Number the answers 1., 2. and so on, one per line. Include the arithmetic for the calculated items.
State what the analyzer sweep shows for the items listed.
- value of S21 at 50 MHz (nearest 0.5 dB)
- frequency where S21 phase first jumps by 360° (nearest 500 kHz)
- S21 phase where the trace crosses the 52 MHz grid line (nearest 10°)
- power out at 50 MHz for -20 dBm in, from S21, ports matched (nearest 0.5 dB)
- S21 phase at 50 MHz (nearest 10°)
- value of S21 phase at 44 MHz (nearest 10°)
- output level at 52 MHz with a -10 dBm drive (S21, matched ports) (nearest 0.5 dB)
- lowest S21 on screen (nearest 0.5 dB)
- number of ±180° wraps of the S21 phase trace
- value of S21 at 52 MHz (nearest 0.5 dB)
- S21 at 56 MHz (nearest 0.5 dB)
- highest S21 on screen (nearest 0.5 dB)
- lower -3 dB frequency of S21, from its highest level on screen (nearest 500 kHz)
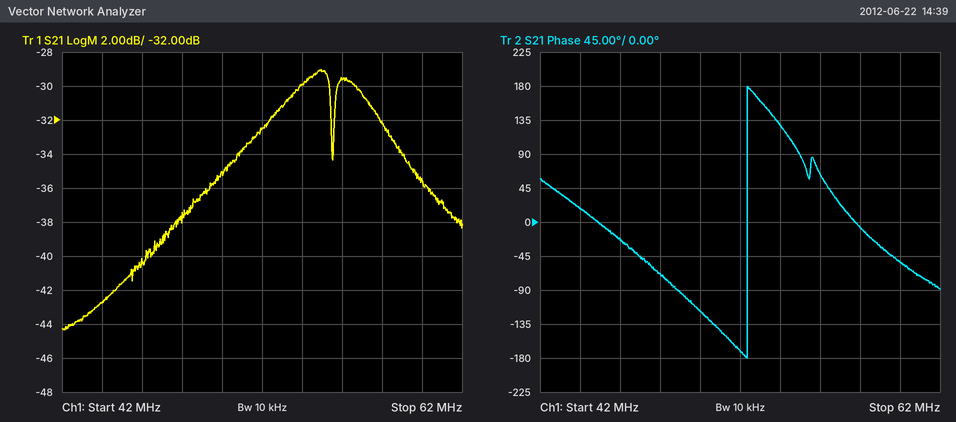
1. -35.0 dB
2. 52.5 MHz
3. -170°
4. -20 dBm + (-35.0 dB) = -55.0 dBm
5. -120°
6. 20°
7. -10 dBm + (-32.5 dB) = -42.5 dBm
8. -44.5 dB
9. 1
10. -32.5 dB
11. -29.5 dB
12. -29.0 dB
13. 52.5 MHz
